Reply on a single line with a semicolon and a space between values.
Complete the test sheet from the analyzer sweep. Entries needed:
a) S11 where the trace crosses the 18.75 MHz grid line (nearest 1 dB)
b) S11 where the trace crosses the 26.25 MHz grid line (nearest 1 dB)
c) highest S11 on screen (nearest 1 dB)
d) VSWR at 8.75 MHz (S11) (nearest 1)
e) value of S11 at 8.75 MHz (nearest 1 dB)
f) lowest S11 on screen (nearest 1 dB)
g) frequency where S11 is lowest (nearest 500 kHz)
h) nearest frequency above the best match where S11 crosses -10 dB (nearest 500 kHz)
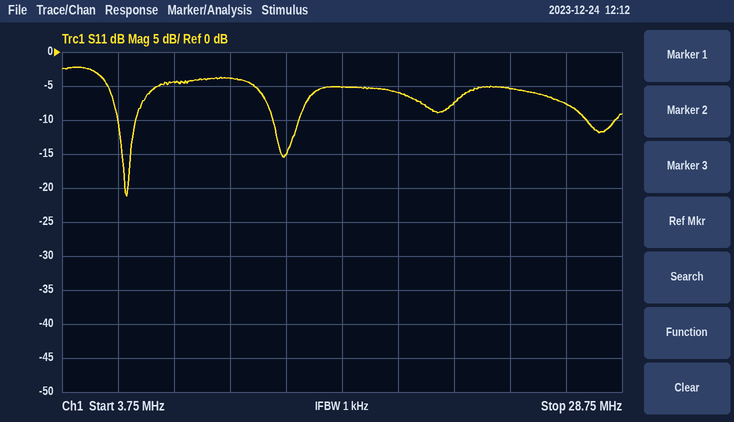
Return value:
-6 dB; -8 dB; -2 dB; 4; -4 dB; -21 dB; 6.5 MHz; 7.0 MHz
